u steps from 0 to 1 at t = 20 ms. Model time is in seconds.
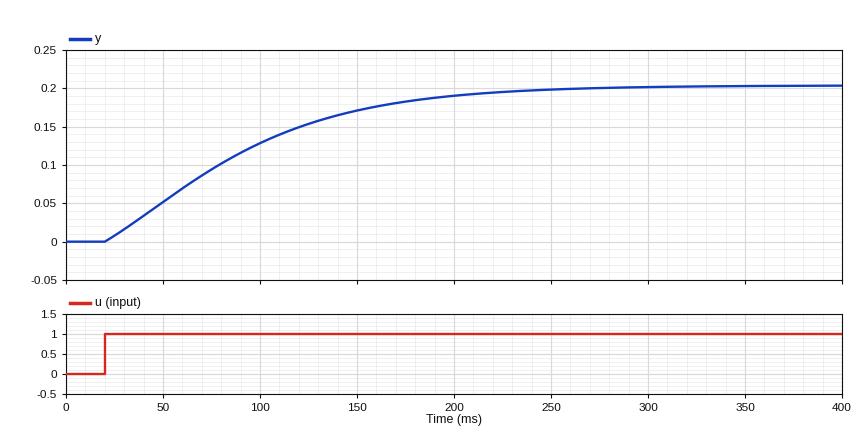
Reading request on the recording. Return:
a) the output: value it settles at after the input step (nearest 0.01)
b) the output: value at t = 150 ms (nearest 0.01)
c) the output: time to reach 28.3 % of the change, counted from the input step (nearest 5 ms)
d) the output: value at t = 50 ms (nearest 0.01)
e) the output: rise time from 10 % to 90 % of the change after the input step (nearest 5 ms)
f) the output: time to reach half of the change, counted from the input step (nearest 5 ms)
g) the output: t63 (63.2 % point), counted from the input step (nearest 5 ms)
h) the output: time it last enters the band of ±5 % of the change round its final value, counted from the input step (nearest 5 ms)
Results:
0.20
0.17
35 ms
0.05
145 ms
60 ms
80 ms
195 ms
